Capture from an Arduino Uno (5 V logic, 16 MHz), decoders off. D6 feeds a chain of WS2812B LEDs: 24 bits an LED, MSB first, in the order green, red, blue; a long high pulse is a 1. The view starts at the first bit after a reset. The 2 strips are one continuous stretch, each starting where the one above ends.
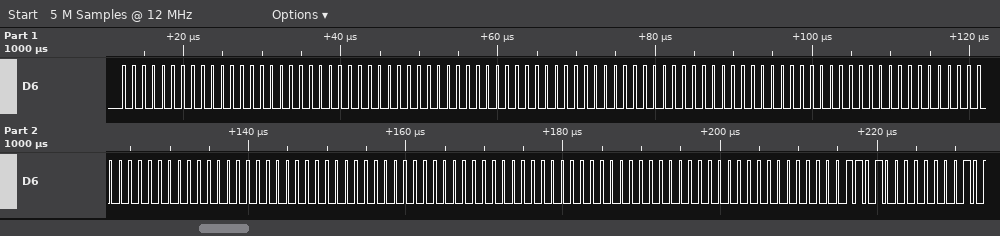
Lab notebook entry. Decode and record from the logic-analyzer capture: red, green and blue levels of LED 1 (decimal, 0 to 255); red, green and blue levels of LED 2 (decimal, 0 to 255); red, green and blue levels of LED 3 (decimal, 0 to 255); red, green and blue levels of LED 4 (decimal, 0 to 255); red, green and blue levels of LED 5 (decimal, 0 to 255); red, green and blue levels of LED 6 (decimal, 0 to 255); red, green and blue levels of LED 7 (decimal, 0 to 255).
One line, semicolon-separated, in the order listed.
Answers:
0, 0, 0; 0, 0, 0; 0, 0, 0; 0, 0, 0; 0, 0, 0; 0, 0, 0; 0, 0, 26
